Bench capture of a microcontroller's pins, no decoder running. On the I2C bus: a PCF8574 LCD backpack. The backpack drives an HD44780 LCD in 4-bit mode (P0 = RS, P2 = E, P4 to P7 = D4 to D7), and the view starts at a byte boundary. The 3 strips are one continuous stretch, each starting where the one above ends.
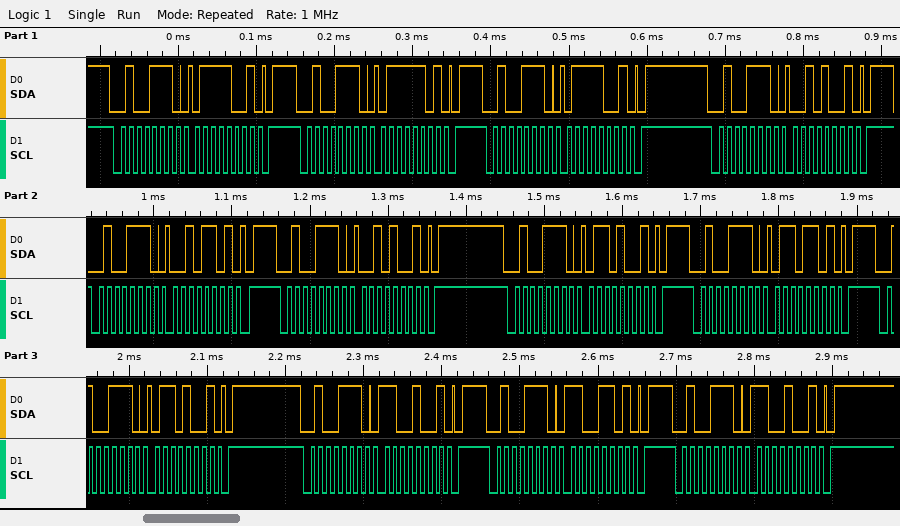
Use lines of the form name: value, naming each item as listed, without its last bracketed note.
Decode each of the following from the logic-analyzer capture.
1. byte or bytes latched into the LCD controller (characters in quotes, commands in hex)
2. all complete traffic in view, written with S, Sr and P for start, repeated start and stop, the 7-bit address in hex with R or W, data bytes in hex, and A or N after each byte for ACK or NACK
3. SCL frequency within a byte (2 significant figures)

byte or bytes latched into the LCD controller: 'r' 'l'
all complete traffic in view, written with S, Sr and P for start, repeated start and stop, the 7-bit address in hex with R or W, data bytes in hex, and A or N after each byte for ACK or NACK: S 27W A 79 A P S 27W A 7D A P S 27W A 79 A P S 27W A 29 A P S 27W A 2D A P S 27W A 29 A P S 27W A 69 A P S 27W A 6D A P S 27W A 69 A P S 27W A C9 A P S 27W A CD A P S 27W A C9 A P
SCL frequency within a byte: 100 kHz
